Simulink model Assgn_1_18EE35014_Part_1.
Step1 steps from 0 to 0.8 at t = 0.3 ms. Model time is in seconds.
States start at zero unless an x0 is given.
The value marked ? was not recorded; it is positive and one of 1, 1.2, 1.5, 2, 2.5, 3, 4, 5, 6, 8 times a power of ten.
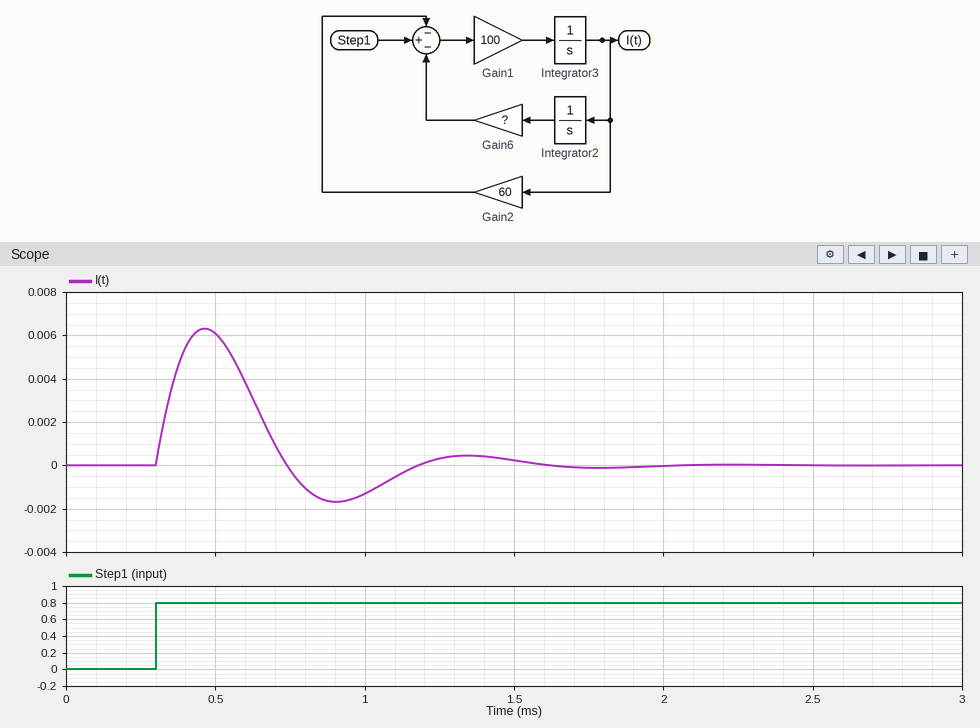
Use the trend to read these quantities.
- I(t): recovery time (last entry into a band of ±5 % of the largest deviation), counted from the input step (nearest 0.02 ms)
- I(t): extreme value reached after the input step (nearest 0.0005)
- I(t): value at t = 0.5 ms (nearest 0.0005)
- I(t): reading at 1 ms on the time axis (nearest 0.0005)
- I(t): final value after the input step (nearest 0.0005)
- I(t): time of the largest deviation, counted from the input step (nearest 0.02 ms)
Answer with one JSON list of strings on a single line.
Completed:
["1.16 ms", "0.0065", "0.0060", "-0.0015", "0.0000", "0.16 ms"]
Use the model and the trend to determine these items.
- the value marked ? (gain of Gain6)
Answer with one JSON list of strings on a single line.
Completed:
["600000"]
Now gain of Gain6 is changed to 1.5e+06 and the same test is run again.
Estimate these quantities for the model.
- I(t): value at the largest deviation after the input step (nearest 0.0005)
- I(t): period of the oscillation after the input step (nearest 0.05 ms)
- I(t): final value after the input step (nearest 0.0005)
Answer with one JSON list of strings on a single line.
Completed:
["0.0045", "0.55 ms", "0.0000"]
